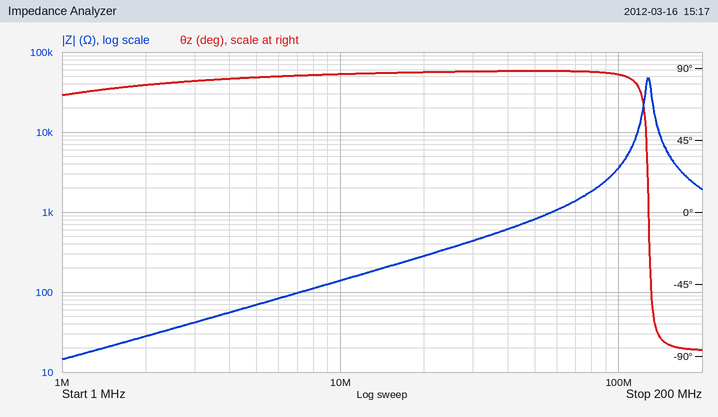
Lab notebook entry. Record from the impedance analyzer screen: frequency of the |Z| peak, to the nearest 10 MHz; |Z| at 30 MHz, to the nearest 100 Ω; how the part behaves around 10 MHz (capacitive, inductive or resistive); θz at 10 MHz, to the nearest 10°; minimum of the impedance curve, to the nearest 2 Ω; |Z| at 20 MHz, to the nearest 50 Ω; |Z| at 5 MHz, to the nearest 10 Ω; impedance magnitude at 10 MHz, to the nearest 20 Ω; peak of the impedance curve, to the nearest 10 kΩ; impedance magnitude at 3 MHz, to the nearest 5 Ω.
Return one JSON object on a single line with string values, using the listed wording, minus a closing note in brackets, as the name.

{"frequency of the |Z| peak, to the nearest 10 MHz": "130 MHz", "|Z| at 30 MHz, to the nearest 100 Ω": "400 Ω", "how the part behaves around 10 MHz": "inductive", "θz at 10 MHz, to the nearest 10°": "90°", "minimum of the impedance curve, to the nearest 2 Ω": "14 Ω", "|Z| at 20 MHz, to the nearest 50 Ω": "300 Ω", "|Z| at 5 MHz, to the nearest 10 Ω": "70 Ω", "impedance magnitude at 10 MHz, to the nearest 20 Ω": "140 Ω", "peak of the impedance curve, to the nearest 10 kΩ": "50 kΩ", "impedance magnitude at 3 MHz, to the nearest 5 Ω": "40 Ω"}
